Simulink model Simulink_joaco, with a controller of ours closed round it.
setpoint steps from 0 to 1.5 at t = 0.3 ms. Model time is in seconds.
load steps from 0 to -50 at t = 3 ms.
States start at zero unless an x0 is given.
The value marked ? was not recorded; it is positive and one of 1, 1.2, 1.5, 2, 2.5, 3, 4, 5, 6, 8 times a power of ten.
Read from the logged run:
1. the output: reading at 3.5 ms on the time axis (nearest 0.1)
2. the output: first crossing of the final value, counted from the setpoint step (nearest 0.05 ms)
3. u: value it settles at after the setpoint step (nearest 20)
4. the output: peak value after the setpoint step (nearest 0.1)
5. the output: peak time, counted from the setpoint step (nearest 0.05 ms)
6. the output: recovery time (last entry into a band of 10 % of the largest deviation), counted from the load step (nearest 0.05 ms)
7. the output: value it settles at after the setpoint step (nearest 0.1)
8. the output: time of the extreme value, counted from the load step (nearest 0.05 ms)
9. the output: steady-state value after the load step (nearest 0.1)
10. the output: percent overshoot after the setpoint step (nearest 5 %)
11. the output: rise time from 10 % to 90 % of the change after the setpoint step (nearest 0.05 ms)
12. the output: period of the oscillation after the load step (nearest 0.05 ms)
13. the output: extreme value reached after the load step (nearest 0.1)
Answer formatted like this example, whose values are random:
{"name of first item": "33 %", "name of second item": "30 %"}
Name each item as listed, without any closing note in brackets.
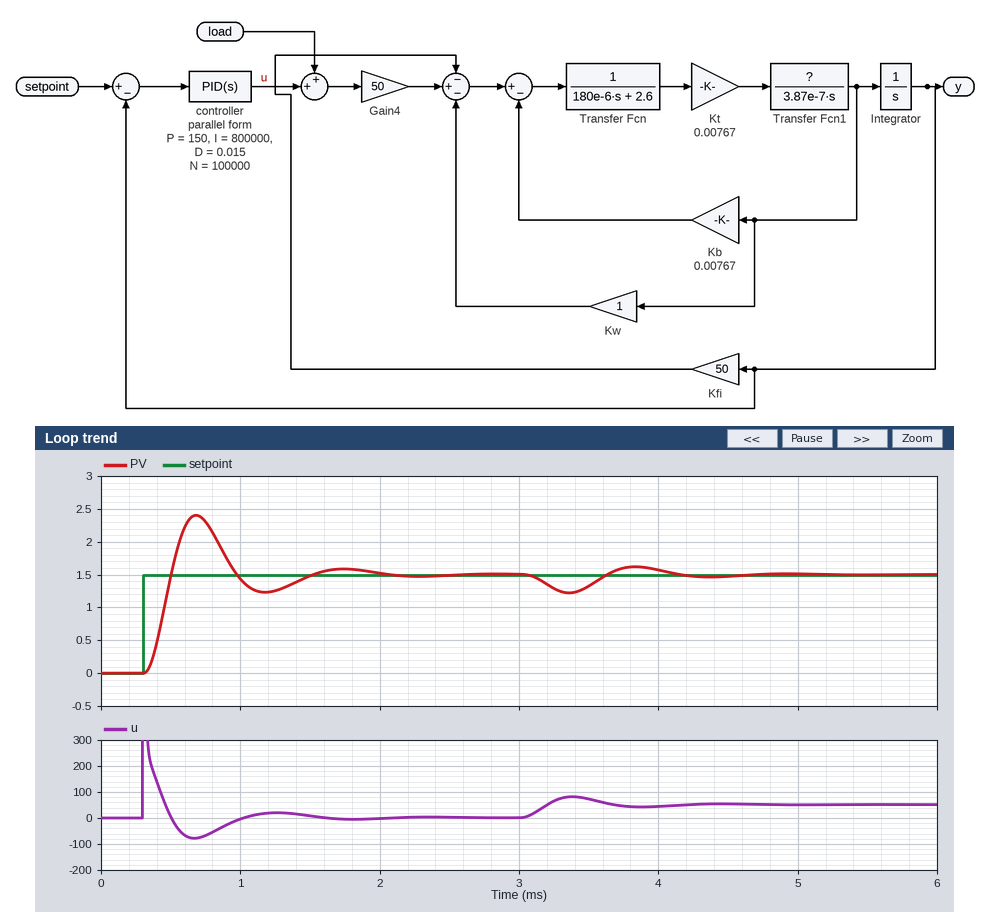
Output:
{"the output: reading at 3.5 ms on the time axis": "1.3", "the output: first crossing of the final value, counted from the setpoint step": "0.20 ms", "u: value it settles at after the setpoint step": "0", "the output: peak value after the setpoint step": "2.4", "the output: peak time, counted from the setpoint step": "0.40 ms", "the output: recovery time (last entry into a band of 10 % of the largest deviation), counted from the load step": "1.50 ms", "the output: value it settles at after the setpoint step": "1.5", "the output: time of the extreme value, counted from the load step": "0.35 ms", "the output: steady-state value after the load step": "1.5", "the output: percent overshoot after the setpoint step": "60 %", "the output: rise time from 10 % to 90 % of the change after the setpoint step": "0.15 ms", "the output: period of the oscillation after the load step": "1.00 ms", "the output: extreme value reached after the load step": "1.2"}
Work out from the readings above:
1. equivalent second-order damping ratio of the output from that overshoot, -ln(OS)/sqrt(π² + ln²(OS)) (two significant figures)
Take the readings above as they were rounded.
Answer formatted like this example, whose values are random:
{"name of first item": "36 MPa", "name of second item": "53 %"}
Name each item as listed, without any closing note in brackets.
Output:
{"equivalent second-order damping ratio of the output from that overshoot, -ln(OS)/sqrt(π² + ln²(OS))": "0.16"}
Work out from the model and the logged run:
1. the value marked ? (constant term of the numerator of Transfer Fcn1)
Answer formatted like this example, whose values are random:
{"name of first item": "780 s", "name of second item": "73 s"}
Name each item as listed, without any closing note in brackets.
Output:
{"the value marked ?": "1"}
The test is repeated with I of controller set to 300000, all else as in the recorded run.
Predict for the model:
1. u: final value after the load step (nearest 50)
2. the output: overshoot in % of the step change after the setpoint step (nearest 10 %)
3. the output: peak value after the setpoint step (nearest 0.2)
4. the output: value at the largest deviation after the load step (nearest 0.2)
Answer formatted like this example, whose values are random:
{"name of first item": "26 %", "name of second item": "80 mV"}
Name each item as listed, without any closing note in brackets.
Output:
{"u: final value after the load step": "50", "the output: overshoot in % of the step change after the setpoint step": "30 %", "the output: peak value after the setpoint step": "2.0", "the output: value at the largest deviation after the load step": "1.2"}
